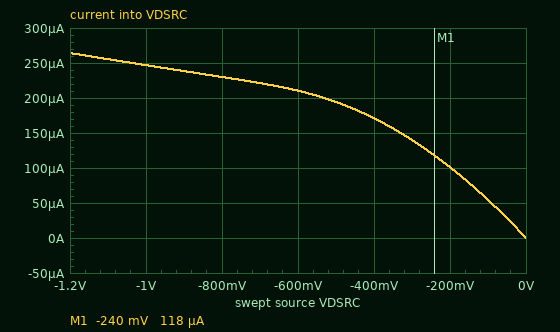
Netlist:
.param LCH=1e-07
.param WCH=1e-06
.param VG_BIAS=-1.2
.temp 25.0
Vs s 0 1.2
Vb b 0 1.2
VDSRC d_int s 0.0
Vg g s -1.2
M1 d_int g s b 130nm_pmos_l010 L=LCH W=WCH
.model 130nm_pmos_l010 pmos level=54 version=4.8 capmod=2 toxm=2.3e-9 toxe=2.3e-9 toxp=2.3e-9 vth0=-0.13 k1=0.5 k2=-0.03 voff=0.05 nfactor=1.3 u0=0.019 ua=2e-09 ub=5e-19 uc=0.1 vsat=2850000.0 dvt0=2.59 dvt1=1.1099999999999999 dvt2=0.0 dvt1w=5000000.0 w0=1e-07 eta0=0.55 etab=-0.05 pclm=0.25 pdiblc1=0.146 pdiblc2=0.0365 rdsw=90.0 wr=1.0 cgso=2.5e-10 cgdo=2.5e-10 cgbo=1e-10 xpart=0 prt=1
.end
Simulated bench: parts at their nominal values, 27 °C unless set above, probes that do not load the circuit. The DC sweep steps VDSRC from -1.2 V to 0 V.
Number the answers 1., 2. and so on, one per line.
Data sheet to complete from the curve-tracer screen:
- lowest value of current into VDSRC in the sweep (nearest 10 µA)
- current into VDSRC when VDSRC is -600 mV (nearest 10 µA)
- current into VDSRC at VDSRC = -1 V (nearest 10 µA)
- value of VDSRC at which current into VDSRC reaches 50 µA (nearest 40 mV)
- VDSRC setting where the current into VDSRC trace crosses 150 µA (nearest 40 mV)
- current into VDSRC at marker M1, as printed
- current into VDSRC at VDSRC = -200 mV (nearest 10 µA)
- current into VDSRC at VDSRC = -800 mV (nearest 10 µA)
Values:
1. 0 A
2. 210 µA
3. 250 µA
4. -80 mV
5. -320 mV
6. 118 µA
7. 100 µA
8. 230 µA
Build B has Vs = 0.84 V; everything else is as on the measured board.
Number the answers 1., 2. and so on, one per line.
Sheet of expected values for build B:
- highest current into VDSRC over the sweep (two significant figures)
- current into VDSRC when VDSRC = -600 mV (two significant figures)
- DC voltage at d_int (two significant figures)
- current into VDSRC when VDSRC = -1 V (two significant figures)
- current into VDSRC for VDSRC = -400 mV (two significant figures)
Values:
1. 3.9 mA
2. 3.0 mA
3. 840 mV
4. 3.6 mA
5. 2.4 mA
